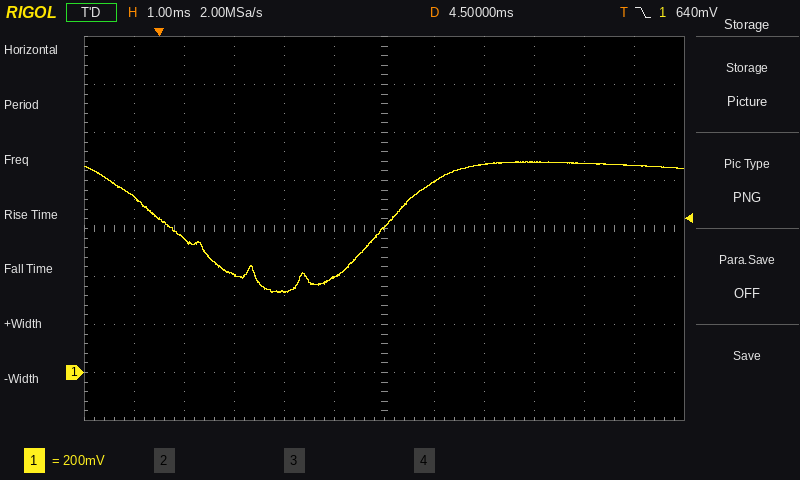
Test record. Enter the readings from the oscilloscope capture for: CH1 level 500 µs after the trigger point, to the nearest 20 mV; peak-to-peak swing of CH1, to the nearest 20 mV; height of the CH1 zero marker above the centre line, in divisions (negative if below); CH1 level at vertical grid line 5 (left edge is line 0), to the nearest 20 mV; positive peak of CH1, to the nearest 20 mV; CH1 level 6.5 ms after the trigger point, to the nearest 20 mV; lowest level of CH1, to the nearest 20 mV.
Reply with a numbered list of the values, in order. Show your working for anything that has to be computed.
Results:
1. 560 mV
2. 880 mV − (340 mV) = 540 mV
3. -3.0 div
4. 400 mV
5. 880 mV
6. 860 mV
7. 340 mV
